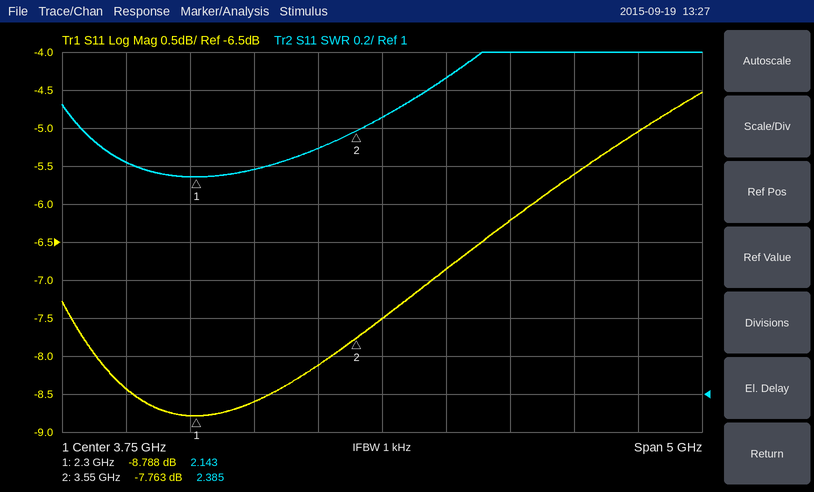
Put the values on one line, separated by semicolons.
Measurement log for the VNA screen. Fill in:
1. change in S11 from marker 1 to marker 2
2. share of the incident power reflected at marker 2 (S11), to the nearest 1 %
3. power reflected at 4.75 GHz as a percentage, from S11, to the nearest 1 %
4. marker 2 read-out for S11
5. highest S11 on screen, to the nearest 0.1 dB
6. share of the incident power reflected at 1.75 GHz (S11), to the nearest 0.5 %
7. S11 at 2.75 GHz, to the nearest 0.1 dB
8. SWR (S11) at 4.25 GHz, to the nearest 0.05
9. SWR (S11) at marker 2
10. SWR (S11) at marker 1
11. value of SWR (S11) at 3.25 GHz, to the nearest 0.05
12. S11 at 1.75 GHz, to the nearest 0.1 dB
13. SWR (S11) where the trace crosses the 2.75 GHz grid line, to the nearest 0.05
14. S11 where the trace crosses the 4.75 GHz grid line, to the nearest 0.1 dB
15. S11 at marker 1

1.025 dB; 17 %; 24 %; -7.763 dB; -4.5 dB; 14.5 %; -8.6 dB; 2.65; 2.385; 2.143; 2.30; -8.4 dB; 2.20; -6.2 dB; -8.788 dB
